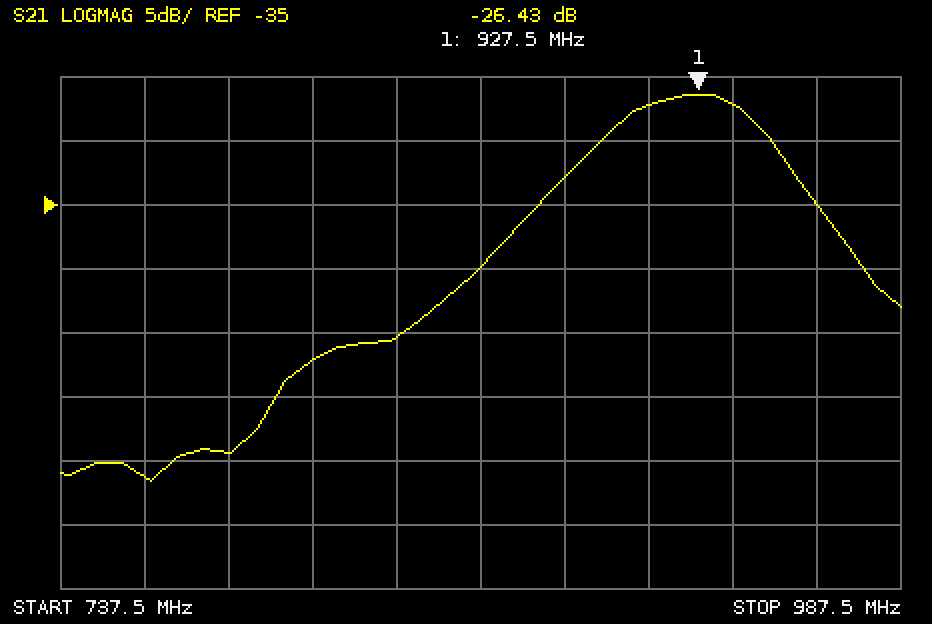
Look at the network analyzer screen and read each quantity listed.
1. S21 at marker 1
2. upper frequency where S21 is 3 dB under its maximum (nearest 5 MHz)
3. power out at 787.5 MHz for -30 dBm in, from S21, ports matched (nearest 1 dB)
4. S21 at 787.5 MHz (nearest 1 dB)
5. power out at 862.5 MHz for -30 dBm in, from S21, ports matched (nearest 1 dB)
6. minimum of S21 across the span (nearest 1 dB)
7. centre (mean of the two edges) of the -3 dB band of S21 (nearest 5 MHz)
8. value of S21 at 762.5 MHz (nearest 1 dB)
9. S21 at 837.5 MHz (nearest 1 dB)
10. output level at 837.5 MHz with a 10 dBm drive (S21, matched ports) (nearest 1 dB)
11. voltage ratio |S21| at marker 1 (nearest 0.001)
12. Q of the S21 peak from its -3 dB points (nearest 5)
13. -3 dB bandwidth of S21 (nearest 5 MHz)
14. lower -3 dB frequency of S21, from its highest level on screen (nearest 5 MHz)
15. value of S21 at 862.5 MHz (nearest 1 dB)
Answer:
-26.43 dB
945 MHz
-84 dBm
-54 dB
-70 dBm
-57 dB
925 MHz
-56 dB
-45 dB
-35 dBm
0.048
20
45 MHz
900 MHz
-40 dB
